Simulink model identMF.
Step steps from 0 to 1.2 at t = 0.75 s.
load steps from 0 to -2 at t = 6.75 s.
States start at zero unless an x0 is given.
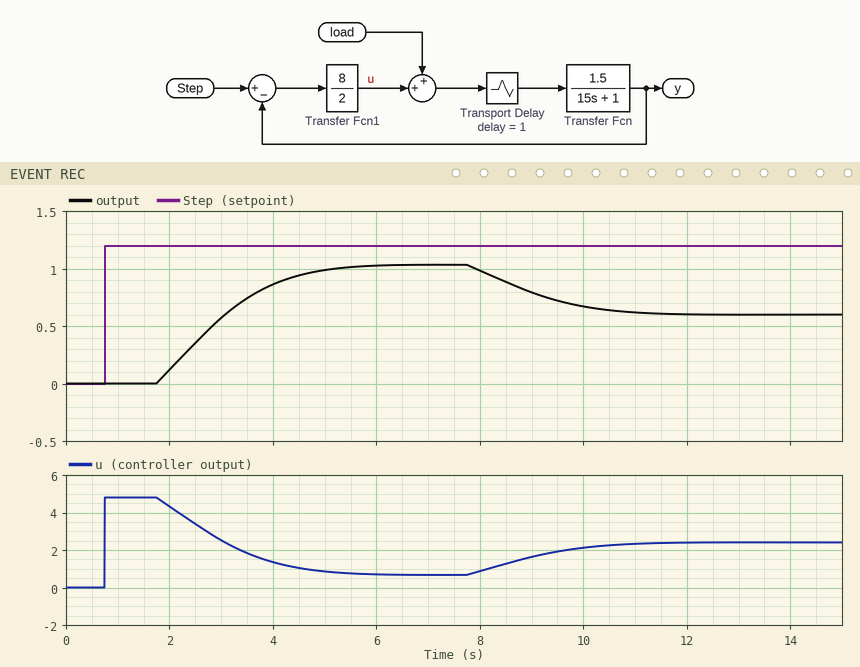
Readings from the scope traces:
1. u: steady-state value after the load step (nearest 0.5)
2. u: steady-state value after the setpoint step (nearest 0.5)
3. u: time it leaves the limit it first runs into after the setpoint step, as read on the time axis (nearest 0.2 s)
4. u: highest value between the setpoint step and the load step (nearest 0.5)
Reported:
2.5
0.5
1.8 s
5.0
